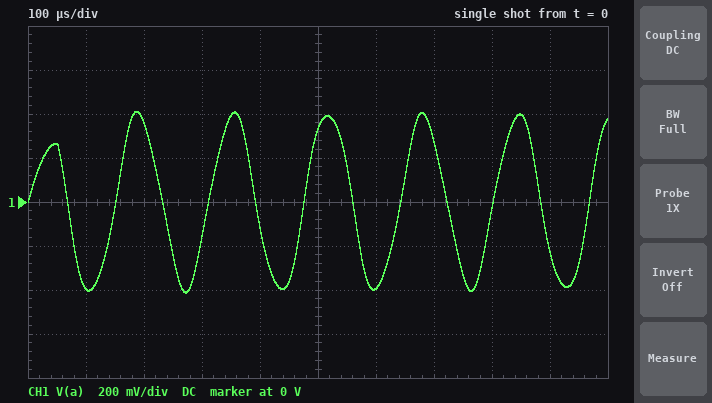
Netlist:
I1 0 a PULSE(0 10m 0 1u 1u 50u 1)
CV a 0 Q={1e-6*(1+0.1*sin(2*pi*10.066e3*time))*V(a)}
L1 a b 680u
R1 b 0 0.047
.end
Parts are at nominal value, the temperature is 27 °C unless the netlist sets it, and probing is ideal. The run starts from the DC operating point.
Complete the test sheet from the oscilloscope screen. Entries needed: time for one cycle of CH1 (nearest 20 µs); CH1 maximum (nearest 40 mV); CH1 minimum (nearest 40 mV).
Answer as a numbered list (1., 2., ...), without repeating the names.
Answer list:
1. 160 µs
2. 400 mV
3. -400 mV
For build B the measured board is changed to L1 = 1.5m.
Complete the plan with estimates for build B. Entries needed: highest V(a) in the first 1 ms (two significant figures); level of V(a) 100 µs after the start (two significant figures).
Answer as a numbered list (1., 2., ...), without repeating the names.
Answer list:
1. 580 mV
2. -150 mV
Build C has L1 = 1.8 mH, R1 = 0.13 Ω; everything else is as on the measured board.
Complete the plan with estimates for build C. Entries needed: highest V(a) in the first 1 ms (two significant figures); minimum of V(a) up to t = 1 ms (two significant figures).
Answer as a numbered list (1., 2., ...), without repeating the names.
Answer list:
1. 540 mV
2. -550 mV
